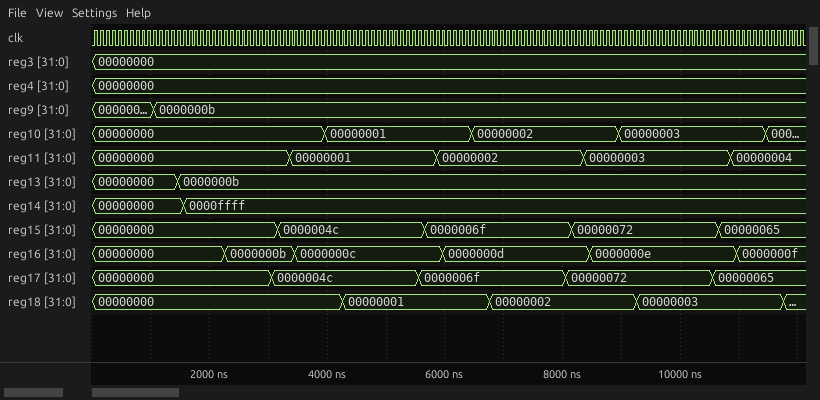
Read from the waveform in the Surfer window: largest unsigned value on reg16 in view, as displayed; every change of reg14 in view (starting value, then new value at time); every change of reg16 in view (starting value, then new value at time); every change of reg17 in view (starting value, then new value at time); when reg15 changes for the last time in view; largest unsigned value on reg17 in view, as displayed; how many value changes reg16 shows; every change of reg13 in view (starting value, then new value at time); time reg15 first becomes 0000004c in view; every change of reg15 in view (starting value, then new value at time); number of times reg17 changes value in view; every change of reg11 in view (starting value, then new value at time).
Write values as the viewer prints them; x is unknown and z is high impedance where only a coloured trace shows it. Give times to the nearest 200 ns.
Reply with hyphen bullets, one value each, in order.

- 0000000f
- 00000000, 0000ffff at 1600 ns
- 00000000, 0000000b at 2200 ns, 0000000c at 3400 ns, 0000000d at 6000 ns, 0000000e at 8400 ns, 0000000f at 11000 ns
- 00000000, 0000004c at 3000 ns, 0000006f at 5600 ns, 00000072 at 8000 ns, 00000065 at 10600 ns
- 10600 ns
- 00000072
- 5
- 00000000, 0000000b at 1400 ns
- 3200 ns
- 00000000, 0000004c at 3200 ns, 0000006f at 5600 ns, 00000072 at 8200 ns, 00000065 at 10600 ns
- 4
- 00000000, 00000001 at 3400 ns, 00000002 at 5800 ns, 00000003 at 8400 ns, 00000004 at 10800 ns
